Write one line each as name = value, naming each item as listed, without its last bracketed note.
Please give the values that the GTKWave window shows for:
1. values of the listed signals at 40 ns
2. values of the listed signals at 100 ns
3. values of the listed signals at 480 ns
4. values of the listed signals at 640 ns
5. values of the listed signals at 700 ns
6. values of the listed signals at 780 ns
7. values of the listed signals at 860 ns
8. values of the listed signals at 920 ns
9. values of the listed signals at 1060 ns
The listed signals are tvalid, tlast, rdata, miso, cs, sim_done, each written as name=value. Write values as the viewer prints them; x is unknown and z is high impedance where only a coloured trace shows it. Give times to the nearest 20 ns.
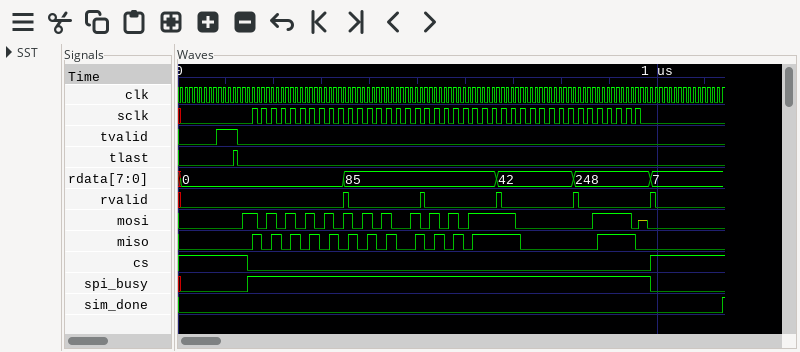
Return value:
values of the listed signals at 40 ns = tvalid=0, tlast=0, rdata=0, miso=0, cs=1, sim_done=0
values of the listed signals at 100 ns = tvalid=1, tlast=0, rdata=0, miso=0, cs=1, sim_done=0
values of the listed signals at 480 ns = tvalid=0, tlast=0, rdata=85, miso=0, cs=0, sim_done=0
values of the listed signals at 640 ns = tvalid=0, tlast=0, rdata=85, miso=1, cs=0, sim_done=0
values of the listed signals at 700 ns = tvalid=0, tlast=0, rdata=42, miso=1, cs=0, sim_done=0
values of the listed signals at 780 ns = tvalid=0, tlast=0, rdata=42, miso=0, cs=0, sim_done=0
values of the listed signals at 860 ns = tvalid=0, tlast=0, rdata=248, miso=0, cs=0, sim_done=0
values of the listed signals at 920 ns = tvalid=0, tlast=0, rdata=248, miso=1, cs=0, sim_done=0
values of the listed signals at 1060 ns = tvalid=0, tlast=0, rdata=7, miso=0, cs=1, sim_done=0
